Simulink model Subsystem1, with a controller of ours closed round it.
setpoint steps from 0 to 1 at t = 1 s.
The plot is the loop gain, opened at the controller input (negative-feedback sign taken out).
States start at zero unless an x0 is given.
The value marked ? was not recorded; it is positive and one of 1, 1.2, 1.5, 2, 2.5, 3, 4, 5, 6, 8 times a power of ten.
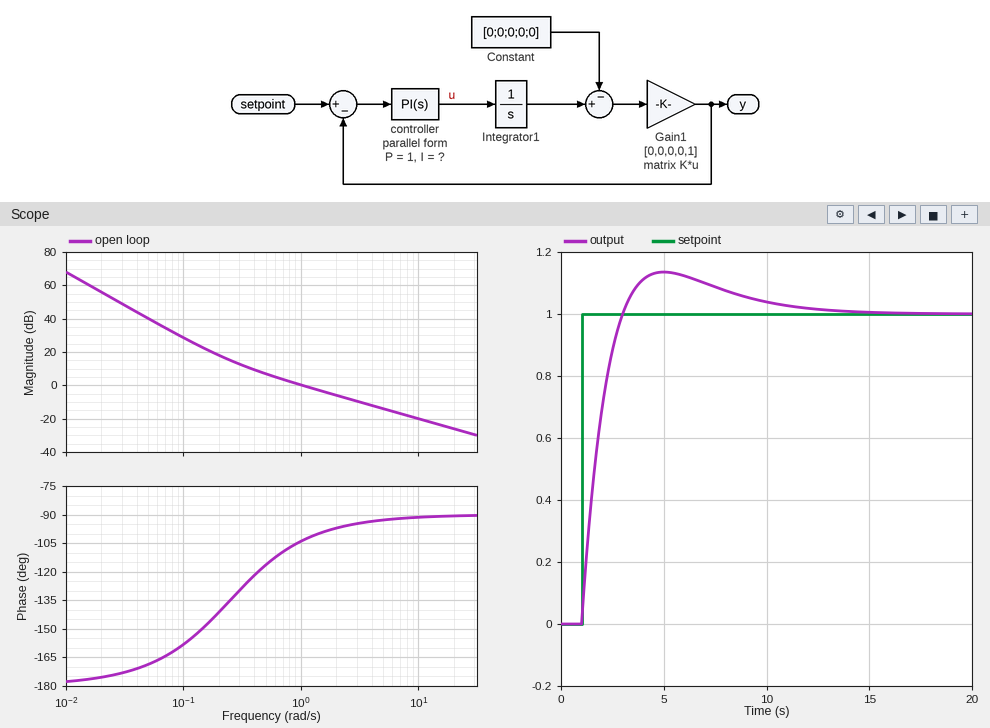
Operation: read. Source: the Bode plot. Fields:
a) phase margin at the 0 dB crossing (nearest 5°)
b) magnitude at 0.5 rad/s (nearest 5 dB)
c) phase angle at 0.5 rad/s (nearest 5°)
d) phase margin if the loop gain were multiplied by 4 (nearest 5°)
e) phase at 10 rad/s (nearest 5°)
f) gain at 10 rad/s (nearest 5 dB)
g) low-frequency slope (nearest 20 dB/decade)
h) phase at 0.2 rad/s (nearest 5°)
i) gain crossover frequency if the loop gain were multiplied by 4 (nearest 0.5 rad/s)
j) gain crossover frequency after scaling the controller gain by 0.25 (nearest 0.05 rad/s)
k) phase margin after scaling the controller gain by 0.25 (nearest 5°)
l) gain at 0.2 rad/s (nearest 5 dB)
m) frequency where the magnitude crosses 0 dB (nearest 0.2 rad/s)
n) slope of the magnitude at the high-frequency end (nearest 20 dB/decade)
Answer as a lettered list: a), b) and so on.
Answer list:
a) 75°
b) 5 dB
c) -115°
d) 85°
e) -90°
f) -20 dB
g) -40 dB/decade
h) -140°
i) 4.0 rad/s
j) 0.30 rad/s
k) 50°
l) 20 dB
m) 1.0 rad/s
n) -20 dB/decade
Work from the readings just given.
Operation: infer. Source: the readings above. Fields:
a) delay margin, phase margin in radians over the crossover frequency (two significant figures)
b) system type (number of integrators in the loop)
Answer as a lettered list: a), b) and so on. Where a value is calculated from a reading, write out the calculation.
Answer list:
a) 75 × π / 180 / 1 = 1.3 s
b) 2
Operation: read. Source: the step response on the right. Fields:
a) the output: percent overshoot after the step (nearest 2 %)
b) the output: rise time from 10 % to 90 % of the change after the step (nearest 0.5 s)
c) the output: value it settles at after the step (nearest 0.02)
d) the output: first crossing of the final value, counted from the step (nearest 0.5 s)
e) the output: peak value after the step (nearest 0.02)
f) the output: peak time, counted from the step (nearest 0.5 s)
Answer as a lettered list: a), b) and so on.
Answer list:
a) 14 %
b) 1.5 s
c) 1.00
d) 2.0 s
e) 1.14
f) 4.0 s
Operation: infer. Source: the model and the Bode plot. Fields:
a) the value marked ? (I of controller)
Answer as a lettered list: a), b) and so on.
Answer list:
a) 0.25
